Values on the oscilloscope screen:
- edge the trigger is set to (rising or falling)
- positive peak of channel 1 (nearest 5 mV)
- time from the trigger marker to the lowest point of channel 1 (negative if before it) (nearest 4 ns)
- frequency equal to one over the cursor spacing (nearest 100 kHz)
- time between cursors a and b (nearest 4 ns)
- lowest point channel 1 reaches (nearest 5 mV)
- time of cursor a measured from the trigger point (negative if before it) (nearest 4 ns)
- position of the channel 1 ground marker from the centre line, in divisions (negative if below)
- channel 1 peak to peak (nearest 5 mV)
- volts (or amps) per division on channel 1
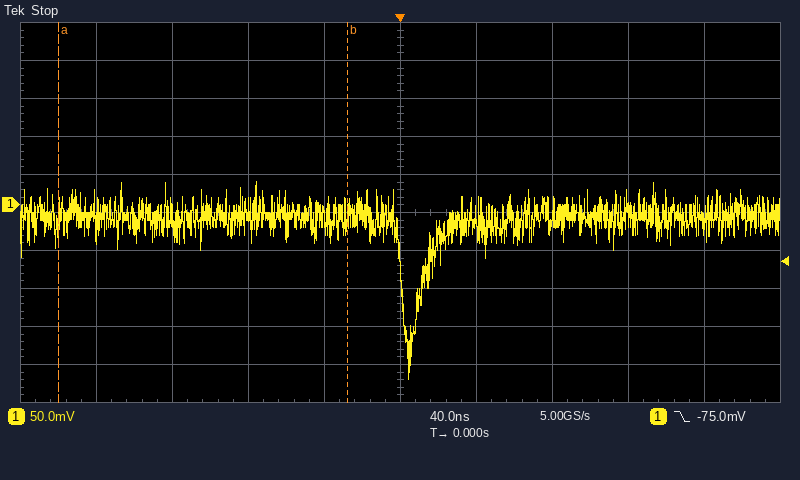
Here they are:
falling
30 mV
+4 ns
6.6 MHz
152 ns
-230 mV
-180 ns
+0.2 div
260 mV
50 mV
